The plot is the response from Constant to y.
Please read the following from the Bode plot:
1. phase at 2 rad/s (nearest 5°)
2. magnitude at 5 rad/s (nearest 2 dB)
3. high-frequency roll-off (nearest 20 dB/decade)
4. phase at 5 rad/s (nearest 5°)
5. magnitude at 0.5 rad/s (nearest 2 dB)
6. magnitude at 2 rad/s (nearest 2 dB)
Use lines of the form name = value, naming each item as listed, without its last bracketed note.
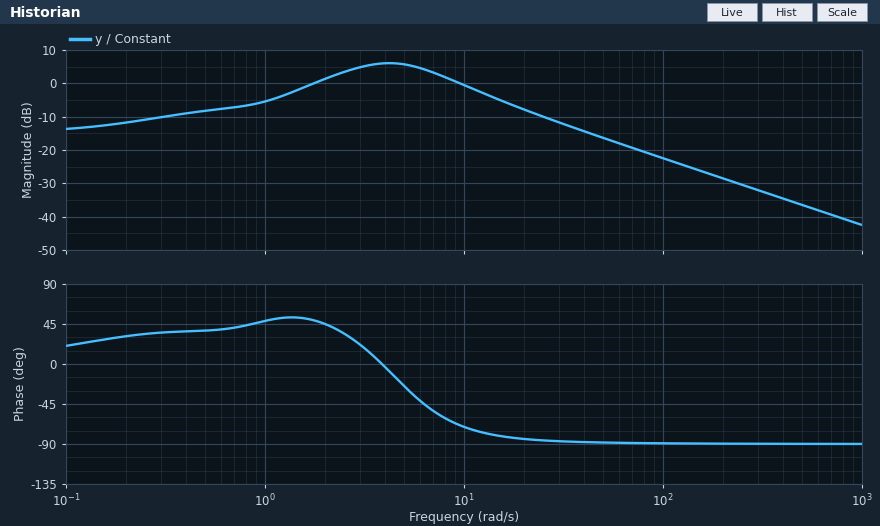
phase at 2 rad/s = 45°
magnitude at 5 rad/s = 6 dB
high-frequency roll-off = -20 dB/decade
phase at 5 rad/s = -25°
magnitude at 0.5 rad/s = -8 dB
magnitude at 2 rad/s = 2 dB
